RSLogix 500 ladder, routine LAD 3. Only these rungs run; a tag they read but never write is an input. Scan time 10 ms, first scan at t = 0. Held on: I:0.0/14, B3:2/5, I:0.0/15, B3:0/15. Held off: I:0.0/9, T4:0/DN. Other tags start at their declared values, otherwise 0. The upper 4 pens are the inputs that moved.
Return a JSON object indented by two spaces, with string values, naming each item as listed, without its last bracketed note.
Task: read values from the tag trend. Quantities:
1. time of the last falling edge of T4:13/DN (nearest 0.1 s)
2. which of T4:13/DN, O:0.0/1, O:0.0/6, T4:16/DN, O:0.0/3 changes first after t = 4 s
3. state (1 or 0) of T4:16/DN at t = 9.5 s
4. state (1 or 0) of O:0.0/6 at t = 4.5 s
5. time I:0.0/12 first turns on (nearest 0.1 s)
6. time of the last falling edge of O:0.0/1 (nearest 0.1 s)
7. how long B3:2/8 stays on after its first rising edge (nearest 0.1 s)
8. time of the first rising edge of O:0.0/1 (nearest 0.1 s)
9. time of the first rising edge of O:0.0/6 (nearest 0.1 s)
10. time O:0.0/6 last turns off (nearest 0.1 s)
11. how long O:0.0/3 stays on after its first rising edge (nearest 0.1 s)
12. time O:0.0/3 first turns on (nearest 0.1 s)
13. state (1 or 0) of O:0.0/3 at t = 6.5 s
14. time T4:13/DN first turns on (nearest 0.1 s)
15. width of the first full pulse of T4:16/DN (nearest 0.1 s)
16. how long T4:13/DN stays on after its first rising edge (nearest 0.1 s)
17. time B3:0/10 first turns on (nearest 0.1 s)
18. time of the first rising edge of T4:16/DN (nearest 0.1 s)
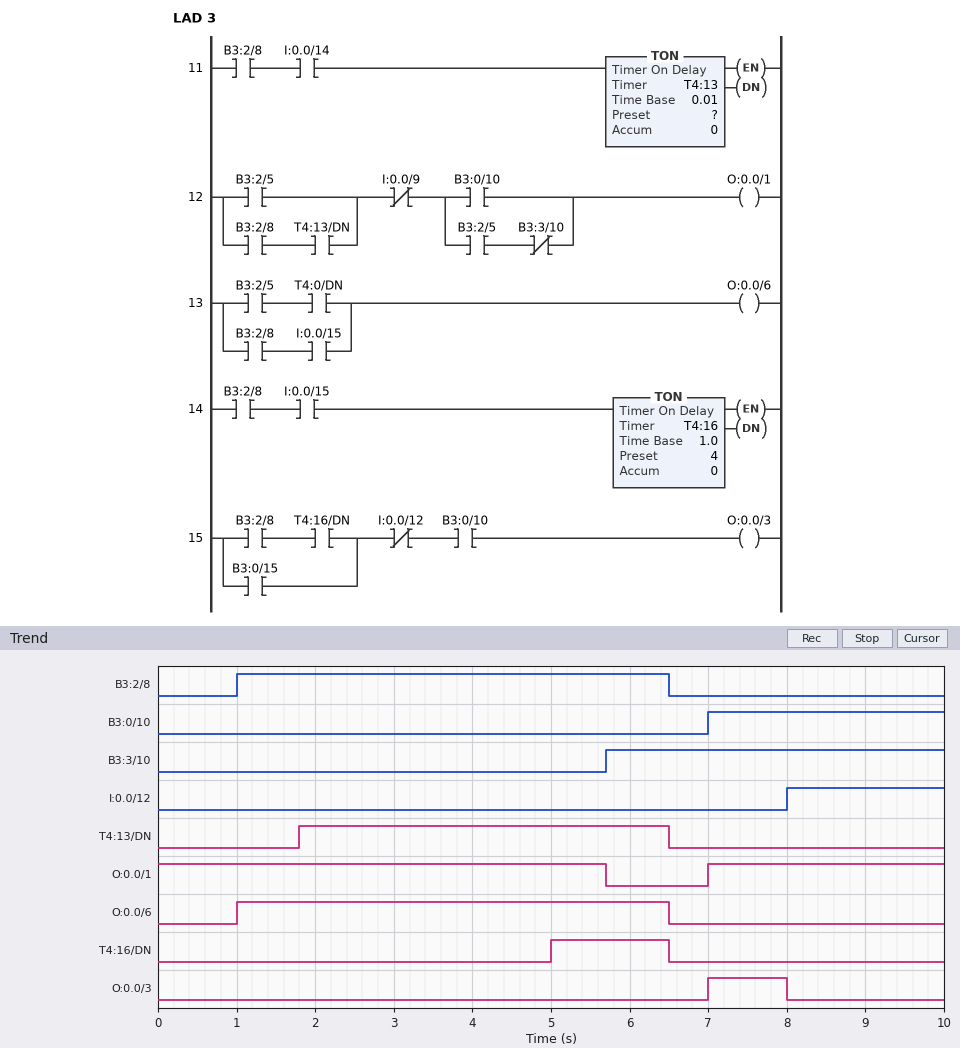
{
  "time of the last falling edge of T4:13/DN": "6.5 s",
  "which of T4:13/DN, O:0.0/1, O:0.0/6, T4:16/DN, O:0.0/3 changes first after t = 4 s": "T4:16/DN",
  "state (1 or 0) of T4:16/DN at t = 9.5 s": "0",
  "state (1 or 0) of O:0.0/6 at t = 4.5 s": "1",
  "time I:0.0/12 first turns on": "8.0 s",
  "time of the last falling edge of O:0.0/1": "5.7 s",
  "how long B3:2/8 stays on after its first rising edge": "5.5 s",
  "time of the first rising edge of O:0.0/1": "7.0 s",
  "time of the first rising edge of O:0.0/6": "1.0 s",
  "time O:0.0/6 last turns off": "6.5 s",
  "how long O:0.0/3 stays on after its first rising edge": "1.0 s",
  "time O:0.0/3 first turns on": "7.0 s",
  "state (1 or 0) of O:0.0/3 at t = 6.5 s": "0",
  "time T4:13/DN first turns on": "1.8 s",
  "width of the first full pulse of T4:16/DN": "1.5 s",
  "how long T4:13/DN stays on after its first rising edge": "4.7 s",
  "time B3:0/10 first turns on": "7.0 s",
  "time of the first rising edge of T4:16/DN": "5.0 s"
}
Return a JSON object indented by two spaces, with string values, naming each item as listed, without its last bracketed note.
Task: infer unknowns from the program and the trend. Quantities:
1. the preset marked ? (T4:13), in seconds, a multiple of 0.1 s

{
  "the preset marked ? (T4:13), in seconds, a multiple of 0.1 s": "0.8 s"
}
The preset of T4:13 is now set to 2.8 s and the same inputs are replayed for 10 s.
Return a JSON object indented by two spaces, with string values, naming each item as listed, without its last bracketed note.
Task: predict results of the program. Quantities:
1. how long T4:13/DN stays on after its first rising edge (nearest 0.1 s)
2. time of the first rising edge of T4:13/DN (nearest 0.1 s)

{
  "how long T4:13/DN stays on after its first rising edge": "2.7 s",
  "time of the first rising edge of T4:13/DN": "3.8 s"
}
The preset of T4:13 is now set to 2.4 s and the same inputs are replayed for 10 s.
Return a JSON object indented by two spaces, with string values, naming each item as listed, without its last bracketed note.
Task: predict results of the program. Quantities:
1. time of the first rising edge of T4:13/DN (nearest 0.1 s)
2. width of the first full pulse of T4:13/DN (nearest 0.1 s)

{
  "time of the first rising edge of T4:13/DN": "3.4 s",
  "width of the first full pulse of T4:13/DN": "3.1 s"
}
